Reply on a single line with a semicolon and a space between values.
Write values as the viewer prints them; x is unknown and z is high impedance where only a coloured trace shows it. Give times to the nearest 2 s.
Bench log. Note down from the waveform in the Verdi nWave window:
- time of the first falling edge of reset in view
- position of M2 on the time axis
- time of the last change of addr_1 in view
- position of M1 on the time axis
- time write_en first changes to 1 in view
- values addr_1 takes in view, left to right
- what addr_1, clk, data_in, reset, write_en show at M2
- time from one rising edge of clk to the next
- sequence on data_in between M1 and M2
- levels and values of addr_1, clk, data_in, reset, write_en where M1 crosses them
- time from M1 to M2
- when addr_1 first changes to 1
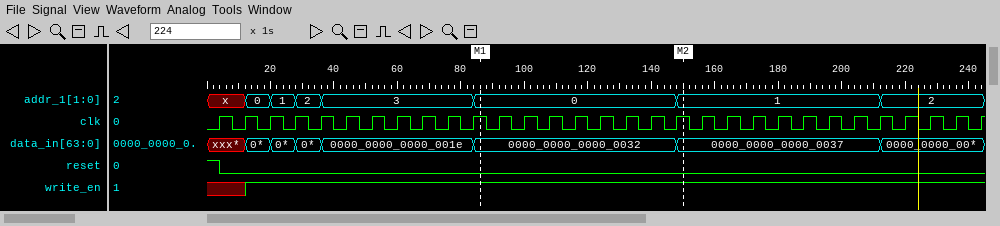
4 s; 150 s; 212 s; 86 s; 12 s; x, 0, 1, 2, 3, 0, 1, 2; addr_1=1, clk=1, data_in=0000_0000_0000_0037, reset=0, write_en=1; 8 s; 0000_0000_0000_0032, 0000_0000_0000_0037; addr_1=0, clk=1, data_in=0000_0000_0000_0032, reset=0, write_en=1; 64 s; 20 s
